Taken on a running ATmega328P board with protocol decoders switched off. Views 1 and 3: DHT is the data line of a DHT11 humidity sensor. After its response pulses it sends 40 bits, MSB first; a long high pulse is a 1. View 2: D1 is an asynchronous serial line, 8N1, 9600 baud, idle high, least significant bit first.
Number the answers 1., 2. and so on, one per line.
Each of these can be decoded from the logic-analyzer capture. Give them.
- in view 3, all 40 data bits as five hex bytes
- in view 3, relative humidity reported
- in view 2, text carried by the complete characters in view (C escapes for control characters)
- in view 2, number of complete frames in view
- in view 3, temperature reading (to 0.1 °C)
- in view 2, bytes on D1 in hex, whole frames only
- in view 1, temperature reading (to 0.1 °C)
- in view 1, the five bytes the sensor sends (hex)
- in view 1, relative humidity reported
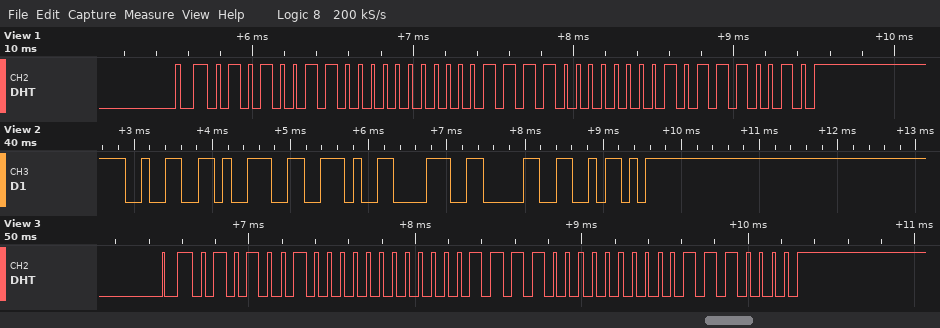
1. 52 00 1E 00 70
2. 82 %
3. "29.80Z"
4. 6
5. 30.0 °C
6. 32 39 2E 38 30 5A
7. 30.1 °C
8. 53 00 1E 01 72
9. 83 %
